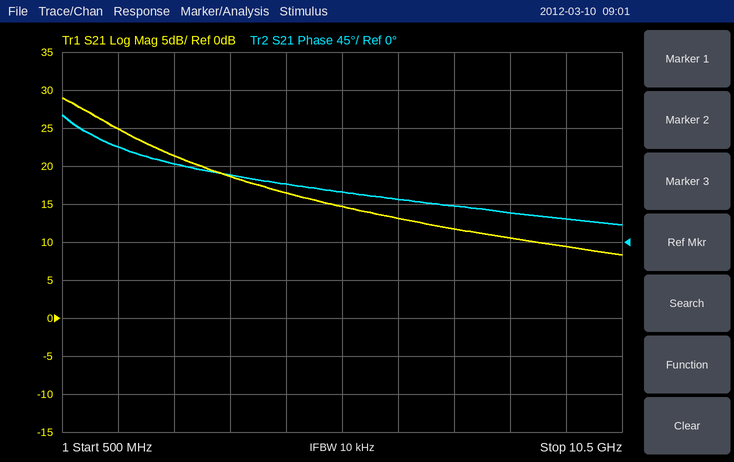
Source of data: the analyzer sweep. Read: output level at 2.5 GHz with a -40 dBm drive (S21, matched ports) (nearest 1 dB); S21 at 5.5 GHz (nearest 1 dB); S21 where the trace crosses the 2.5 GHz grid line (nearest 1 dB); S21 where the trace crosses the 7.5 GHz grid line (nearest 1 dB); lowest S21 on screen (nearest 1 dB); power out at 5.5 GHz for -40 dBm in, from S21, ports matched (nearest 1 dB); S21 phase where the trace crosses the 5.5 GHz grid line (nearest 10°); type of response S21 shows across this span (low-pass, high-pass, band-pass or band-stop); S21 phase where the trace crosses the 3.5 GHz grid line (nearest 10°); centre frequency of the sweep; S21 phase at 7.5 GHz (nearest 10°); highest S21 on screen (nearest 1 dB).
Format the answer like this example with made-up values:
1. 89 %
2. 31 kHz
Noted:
1. -19 dBm
2. 15 dB
3. 21 dB
4. 12 dB
5. 8 dB
6. -25 dBm
7. 60°
8. low-pass
9. 80°
10. 5.5 GHz
11. 40°
12. 29 dB
